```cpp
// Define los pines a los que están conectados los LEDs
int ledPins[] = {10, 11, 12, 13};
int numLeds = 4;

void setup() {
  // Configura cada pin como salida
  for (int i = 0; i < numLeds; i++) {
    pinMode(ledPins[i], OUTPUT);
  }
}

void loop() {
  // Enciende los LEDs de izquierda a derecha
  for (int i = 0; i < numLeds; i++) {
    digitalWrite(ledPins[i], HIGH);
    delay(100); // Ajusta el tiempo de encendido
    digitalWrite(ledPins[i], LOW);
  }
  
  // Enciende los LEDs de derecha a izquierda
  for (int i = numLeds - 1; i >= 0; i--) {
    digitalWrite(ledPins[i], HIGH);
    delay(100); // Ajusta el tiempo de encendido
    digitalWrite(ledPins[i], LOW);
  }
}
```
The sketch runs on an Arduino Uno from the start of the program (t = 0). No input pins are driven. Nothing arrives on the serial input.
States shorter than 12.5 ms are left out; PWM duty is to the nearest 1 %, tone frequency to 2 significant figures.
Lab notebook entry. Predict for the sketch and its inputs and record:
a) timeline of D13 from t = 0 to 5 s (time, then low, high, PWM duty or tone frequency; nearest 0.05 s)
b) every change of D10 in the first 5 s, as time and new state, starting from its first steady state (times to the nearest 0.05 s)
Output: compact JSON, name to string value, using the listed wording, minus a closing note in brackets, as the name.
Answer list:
{"timeline of D13 from t = 0 to 5 s": "0 s low; 0.3 s high; 0.5 s low; 1.1 s high; 1.3 s low; 1.9 s high; 2.1 s low; 2.7 s high; 2.9 s low; 3.5 s high; 3.7 s low; 4.3 s high; 4.5 s low", "every change of D10 in the first 5 s, as time and new state, starting from its first steady state": "0 s high; 0.1 s low; 0.7 s high; 0.9 s low; 1.5 s high; 1.7 s low; 2.3 s high; 2.5 s low; 3.1 s high; 3.3 s low; 3.9 s high; 4.1 s low; 4.7 s high; 4.9 s low"}
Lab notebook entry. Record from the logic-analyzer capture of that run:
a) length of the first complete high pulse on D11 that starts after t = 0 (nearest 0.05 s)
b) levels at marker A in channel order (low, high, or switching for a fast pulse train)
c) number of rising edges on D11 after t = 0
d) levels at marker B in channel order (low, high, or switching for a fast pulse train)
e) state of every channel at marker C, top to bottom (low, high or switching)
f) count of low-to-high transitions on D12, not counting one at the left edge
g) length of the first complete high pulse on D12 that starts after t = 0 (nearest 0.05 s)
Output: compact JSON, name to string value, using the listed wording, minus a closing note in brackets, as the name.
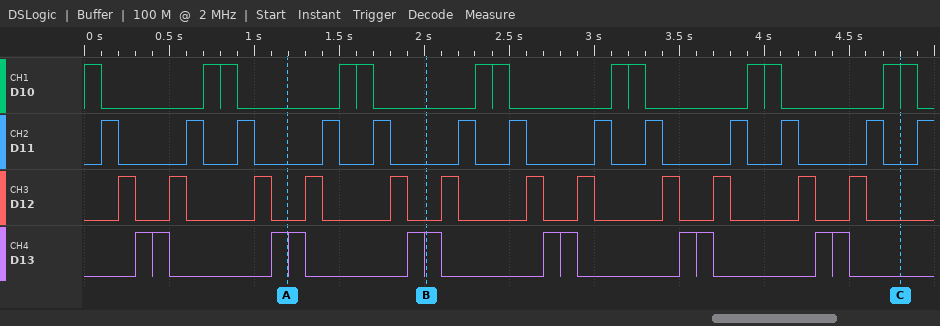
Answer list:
{"length of the first complete high pulse on D11 that starts after t = 0": "0.10 s", "levels at marker A in channel order": "D10 low, D11 low, D12 low, D13 high", "number of rising edges on D11 after t = 0": "13", "levels at marker B in channel order": "D10 low, D11 low, D12 low, D13 high", "state of every channel at marker C, top to bottom": "D10 high, D11 low, D12 low, D13 low", "count of low-to-high transitions on D12, not counting one at the left edge": "12", "length of the first complete high pulse on D12 that starts after t = 0": "0.10 s"}
